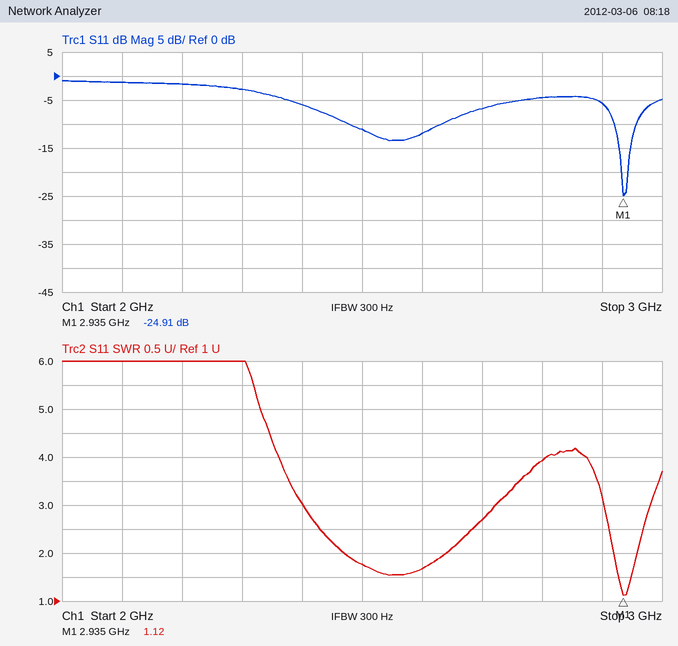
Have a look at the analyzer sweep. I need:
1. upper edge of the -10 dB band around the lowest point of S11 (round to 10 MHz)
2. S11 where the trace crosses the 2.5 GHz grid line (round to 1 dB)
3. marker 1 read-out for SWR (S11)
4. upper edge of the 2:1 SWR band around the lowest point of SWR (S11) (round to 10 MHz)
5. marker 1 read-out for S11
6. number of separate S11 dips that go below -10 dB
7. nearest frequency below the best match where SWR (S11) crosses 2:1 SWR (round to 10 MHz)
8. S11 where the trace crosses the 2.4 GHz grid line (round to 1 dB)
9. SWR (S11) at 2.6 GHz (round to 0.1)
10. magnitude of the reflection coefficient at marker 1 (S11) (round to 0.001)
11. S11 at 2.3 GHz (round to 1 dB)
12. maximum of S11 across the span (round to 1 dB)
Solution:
2.96 GHz
-11 dB
1.12
2.96 GHz
-24.91 dB
2
2.92 GHz
-6 dB
1.7
0.057
-3 dB
-1 dB
